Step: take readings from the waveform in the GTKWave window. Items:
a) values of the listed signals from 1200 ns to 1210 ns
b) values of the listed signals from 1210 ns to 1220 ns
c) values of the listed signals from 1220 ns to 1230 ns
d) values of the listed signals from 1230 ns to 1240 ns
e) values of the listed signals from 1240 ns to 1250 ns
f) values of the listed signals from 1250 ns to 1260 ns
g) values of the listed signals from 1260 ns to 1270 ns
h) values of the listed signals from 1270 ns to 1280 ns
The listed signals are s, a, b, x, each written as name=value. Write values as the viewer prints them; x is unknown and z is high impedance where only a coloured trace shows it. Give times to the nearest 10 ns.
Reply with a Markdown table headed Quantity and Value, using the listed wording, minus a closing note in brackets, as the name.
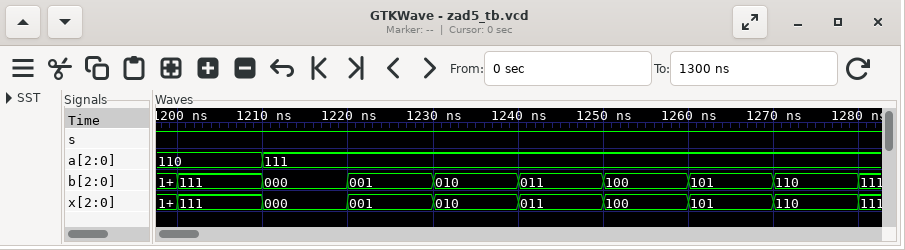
| Quantity | Value |
|---|---|
| values of the listed signals from 1200 ns to 1210 ns | s=1, a=110, b=111, x=111 |
| values of the listed signals from 1210 ns to 1220 ns | s=1, a=111, b=000, x=000 |
| values of the listed signals from 1220 ns to 1230 ns | s=1, a=111, b=001, x=001 |
| values of the listed signals from 1230 ns to 1240 ns | s=1, a=111, b=010, x=010 |
| values of the listed signals from 1240 ns to 1250 ns | s=1, a=111, b=011, x=011 |
| values of the listed signals from 1250 ns to 1260 ns | s=1, a=111, b=100, x=100 |
| values of the listed signals from 1260 ns to 1270 ns | s=1, a=111, b=101, x=101 |
| values of the listed signals from 1270 ns to 1280 ns | s=1, a=111, b=110, x=110 |
